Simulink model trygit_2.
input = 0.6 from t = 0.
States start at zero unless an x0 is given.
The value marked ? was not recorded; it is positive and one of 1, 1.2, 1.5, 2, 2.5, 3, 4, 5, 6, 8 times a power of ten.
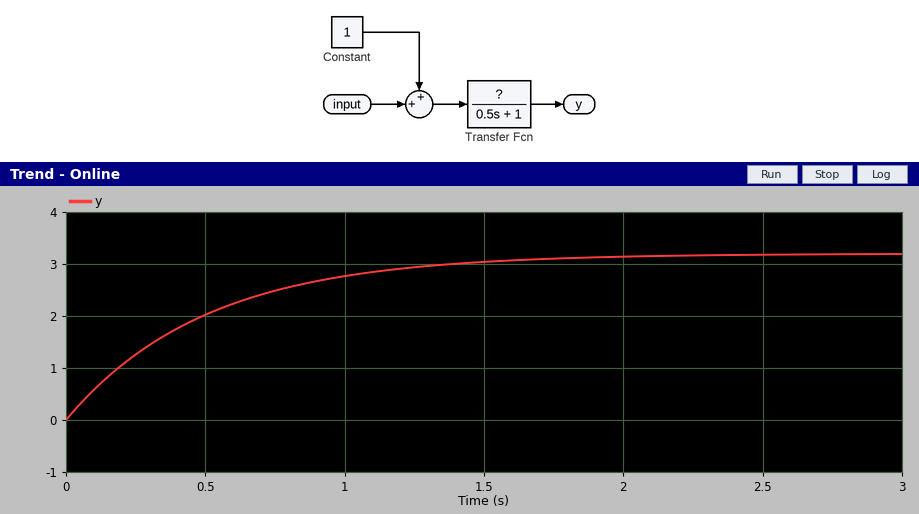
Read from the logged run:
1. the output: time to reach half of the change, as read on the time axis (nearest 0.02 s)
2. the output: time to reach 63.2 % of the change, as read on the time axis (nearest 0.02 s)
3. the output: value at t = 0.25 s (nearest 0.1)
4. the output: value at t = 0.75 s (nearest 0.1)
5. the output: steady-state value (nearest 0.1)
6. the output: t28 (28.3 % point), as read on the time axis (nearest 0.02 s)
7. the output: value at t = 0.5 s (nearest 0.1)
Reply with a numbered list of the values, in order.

1. 0.34 s
2. 0.50 s
3. 1.3
4. 2.5
5. 3.2
6. 0.16 s
7. 2.0
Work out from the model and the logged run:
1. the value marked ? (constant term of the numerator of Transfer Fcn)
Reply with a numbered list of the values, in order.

1. 2
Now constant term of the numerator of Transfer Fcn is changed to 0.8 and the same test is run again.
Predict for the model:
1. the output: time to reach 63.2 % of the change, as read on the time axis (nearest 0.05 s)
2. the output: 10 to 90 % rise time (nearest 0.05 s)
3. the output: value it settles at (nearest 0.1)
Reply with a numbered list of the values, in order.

1. 0.50 s
2. 1.10 s
3. 1.3
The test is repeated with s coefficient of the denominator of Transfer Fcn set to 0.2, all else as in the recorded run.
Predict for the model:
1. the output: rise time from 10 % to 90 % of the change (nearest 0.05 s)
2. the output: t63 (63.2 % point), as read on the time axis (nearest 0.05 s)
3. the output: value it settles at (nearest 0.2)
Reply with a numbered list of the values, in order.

1. 0.45 s
2. 0.20 s
3. 3.2
